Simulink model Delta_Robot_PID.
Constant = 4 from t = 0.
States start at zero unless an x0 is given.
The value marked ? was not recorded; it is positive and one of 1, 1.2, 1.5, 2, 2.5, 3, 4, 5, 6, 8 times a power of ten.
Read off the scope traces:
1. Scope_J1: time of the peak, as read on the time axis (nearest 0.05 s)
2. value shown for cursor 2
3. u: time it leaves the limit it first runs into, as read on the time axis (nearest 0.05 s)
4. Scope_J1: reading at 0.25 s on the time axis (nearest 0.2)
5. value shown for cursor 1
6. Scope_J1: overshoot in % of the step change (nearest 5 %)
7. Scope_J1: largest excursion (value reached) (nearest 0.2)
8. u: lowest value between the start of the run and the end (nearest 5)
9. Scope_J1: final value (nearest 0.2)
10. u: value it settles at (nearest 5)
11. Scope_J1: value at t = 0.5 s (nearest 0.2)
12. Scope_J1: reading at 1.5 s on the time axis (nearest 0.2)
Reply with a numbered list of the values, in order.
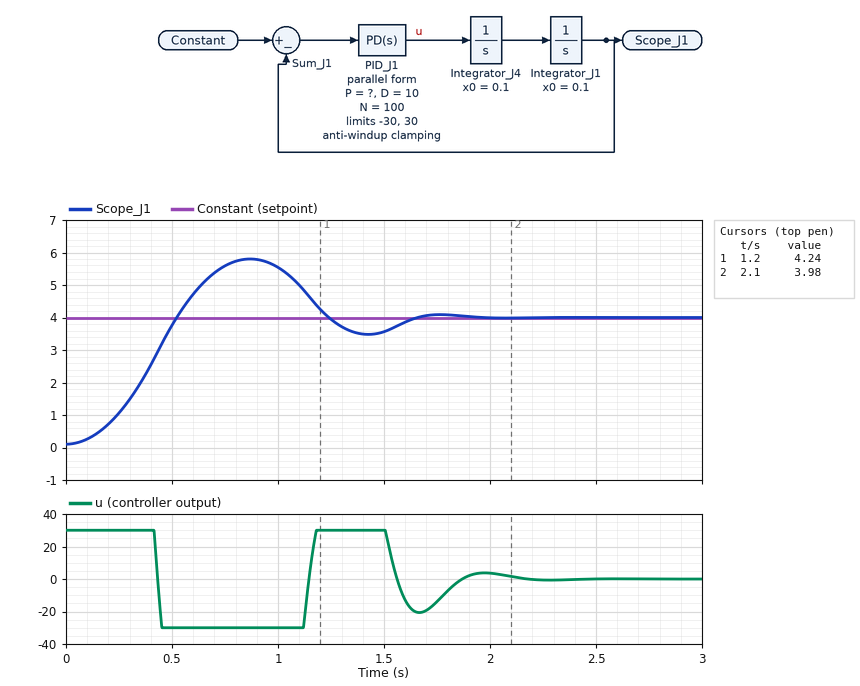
1. 0.85 s
2. 3.98
3. 0.40 s
4. 1.0
5. 4.24
6. 45 %
7. 5.8
8. -30
9. 4.0
10. 0
11. 3.8
12. 3.6
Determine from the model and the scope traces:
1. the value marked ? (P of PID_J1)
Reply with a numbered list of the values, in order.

1. 120
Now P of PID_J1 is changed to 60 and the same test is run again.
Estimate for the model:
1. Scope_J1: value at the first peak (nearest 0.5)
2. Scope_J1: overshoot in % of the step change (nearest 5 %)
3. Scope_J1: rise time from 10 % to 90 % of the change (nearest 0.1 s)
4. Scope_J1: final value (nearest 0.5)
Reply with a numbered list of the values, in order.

1. 4.5
2. 10 %
3. 0.4 s
4. 4.0
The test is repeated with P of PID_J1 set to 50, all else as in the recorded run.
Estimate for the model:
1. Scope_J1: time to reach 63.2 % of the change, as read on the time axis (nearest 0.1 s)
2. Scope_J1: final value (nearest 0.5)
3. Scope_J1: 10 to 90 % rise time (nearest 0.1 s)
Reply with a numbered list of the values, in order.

1. 0.4 s
2. 4.0
3. 0.4 s
